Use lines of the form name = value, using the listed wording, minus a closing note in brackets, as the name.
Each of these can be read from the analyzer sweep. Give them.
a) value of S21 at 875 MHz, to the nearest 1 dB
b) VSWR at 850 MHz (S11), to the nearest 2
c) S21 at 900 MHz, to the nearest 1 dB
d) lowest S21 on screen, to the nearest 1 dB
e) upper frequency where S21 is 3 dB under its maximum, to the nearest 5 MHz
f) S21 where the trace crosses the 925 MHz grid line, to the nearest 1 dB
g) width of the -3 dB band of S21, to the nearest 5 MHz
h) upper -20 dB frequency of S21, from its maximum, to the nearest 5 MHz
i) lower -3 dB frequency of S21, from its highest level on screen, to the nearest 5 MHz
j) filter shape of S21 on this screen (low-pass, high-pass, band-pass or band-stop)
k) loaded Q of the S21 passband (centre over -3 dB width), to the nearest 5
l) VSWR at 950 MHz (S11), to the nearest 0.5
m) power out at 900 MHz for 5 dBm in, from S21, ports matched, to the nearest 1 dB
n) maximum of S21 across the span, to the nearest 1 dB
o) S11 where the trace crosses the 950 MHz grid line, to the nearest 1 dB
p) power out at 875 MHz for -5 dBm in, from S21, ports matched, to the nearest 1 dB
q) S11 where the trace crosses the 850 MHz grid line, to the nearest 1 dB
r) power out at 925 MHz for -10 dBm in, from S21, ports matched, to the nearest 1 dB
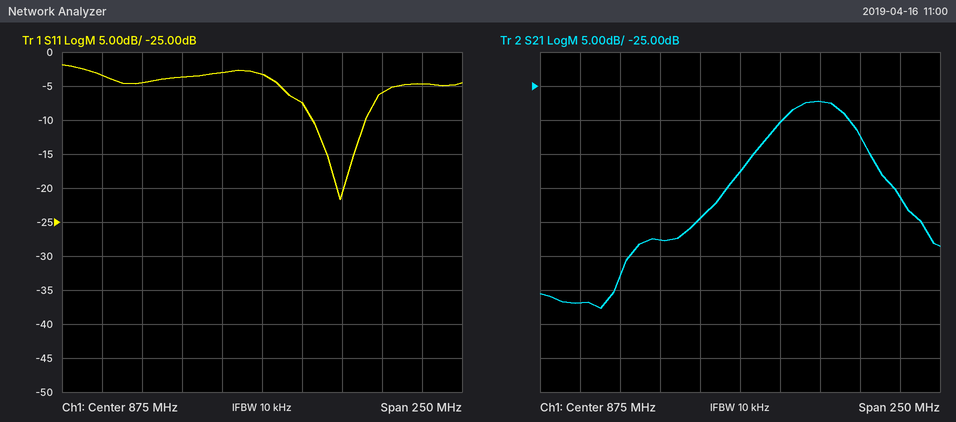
value of S21 at 875 MHz, to the nearest 1 dB = -38 dB
VSWR at 850 MHz (S11), to the nearest 2 = 6
S21 at 900 MHz, to the nearest 1 dB = -30 dB
lowest S21 on screen, to the nearest 1 dB = -58 dB
upper frequency where S21 is 3 dB under its maximum, to the nearest 5 MHz = 945 MHz
S21 where the trace crosses the 925 MHz grid line, to the nearest 1 dB = -27 dB
width of the -3 dB band of S21, to the nearest 5 MHz = 45 MHz
upper -20 dB frequency of S21, from its maximum, to the nearest 5 MHz = 995 MHz
lower -3 dB frequency of S21, from its highest level on screen, to the nearest 5 MHz = 900 MHz
filter shape of S21 on this screen = band-pass
loaded Q of the S21 passband (centre over -3 dB width), to the nearest 5 = 20
VSWR at 950 MHz (S11), to the nearest 0.5 = 3.0
power out at 900 MHz for 5 dBm in, from S21, ports matched, to the nearest 1 dB = -25 dBm
maximum of S21 across the span, to the nearest 1 dB = -27 dB
S11 where the trace crosses the 950 MHz grid line, to the nearest 1 dB = -6 dB
power out at 875 MHz for -5 dBm in, from S21, ports matched, to the nearest 1 dB = -43 dBm
S11 where the trace crosses the 850 MHz grid line, to the nearest 1 dB = -3 dB
power out at 925 MHz for -10 dBm in, from S21, ports matched, to the nearest 1 dB = -37 dBm
